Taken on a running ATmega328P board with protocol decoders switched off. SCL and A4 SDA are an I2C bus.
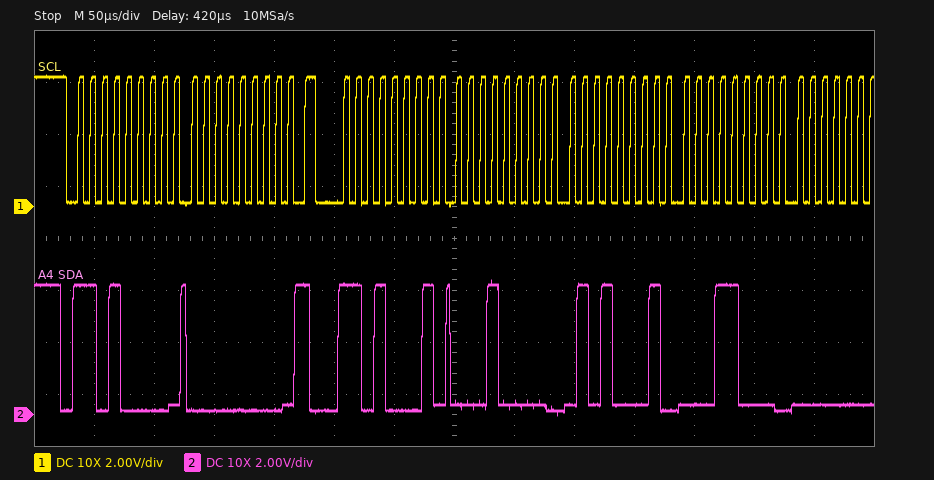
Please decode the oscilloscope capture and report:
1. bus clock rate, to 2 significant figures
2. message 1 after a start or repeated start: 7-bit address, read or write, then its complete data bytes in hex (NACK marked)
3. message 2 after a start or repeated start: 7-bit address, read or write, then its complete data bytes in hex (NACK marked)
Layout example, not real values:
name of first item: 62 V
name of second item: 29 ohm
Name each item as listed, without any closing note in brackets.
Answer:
bus clock rate, to 2 significant figures: 100 kHz
message 1 after a start or repeated start: 7-bit address, read or write, then its complete data bytes in hex: 0x68 write: 00
message 2 after a start or repeated start: 7-bit address, read or write, then its complete data bytes in hex: 0x68 read: 10 51 18
